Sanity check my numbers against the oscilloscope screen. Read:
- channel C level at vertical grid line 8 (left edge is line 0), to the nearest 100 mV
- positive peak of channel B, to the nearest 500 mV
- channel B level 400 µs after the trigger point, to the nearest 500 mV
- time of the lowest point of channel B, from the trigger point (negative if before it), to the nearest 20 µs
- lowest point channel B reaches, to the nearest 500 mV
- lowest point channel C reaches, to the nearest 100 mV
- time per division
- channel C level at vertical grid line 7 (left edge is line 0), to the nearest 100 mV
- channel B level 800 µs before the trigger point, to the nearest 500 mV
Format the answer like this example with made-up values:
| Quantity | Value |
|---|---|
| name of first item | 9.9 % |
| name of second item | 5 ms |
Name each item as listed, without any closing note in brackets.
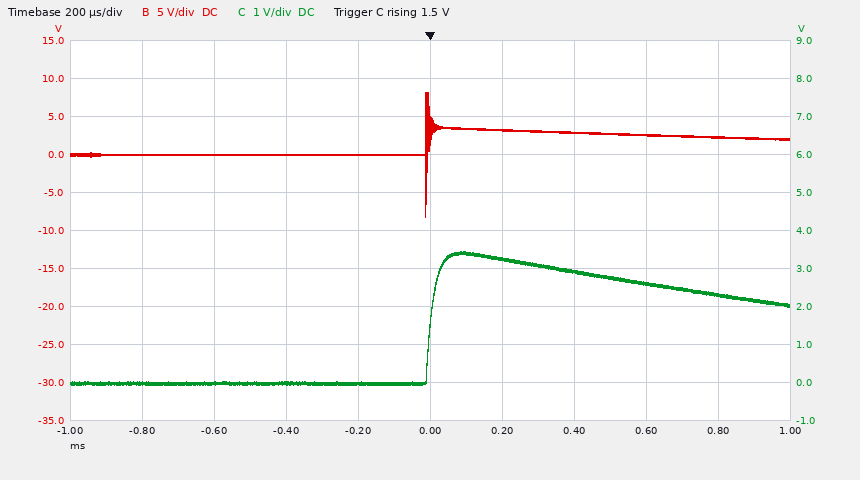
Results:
| Quantity | Value |
|---|---|
| channel C level at vertical grid line 8 (left edge is line 0), to the nearest 100 mV | 2.6 V |
| positive peak of channel B, to the nearest 500 mV | 8.0 V |
| channel B level 400 µs after the trigger point, to the nearest 500 mV | 3.0 V |
| time of the lowest point of channel B, from the trigger point (negative if before it), to the nearest 20 µs | -20 µs |
| lowest point channel B reaches, to the nearest 500 mV | -8.0 V |
| lowest point channel C reaches, to the nearest 100 mV | -100 mV |
| time per division | 200 µs |
| channel C level at vertical grid line 7 (left edge is line 0), to the nearest 100 mV | 2.9 V |
| channel B level 800 µs before the trigger point, to the nearest 500 mV | 0.0 V |
